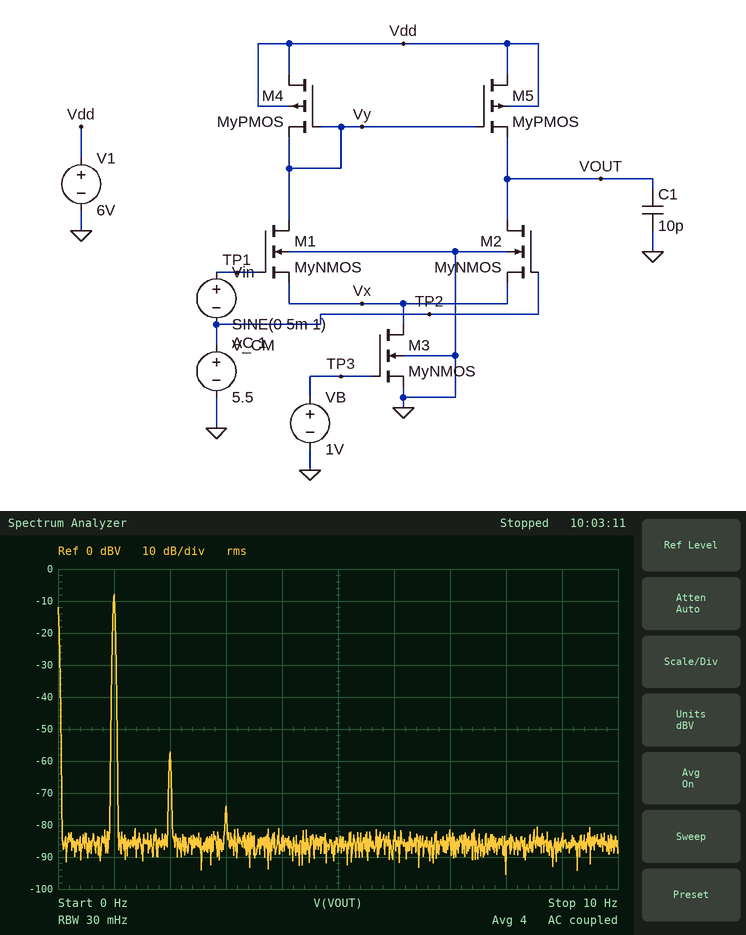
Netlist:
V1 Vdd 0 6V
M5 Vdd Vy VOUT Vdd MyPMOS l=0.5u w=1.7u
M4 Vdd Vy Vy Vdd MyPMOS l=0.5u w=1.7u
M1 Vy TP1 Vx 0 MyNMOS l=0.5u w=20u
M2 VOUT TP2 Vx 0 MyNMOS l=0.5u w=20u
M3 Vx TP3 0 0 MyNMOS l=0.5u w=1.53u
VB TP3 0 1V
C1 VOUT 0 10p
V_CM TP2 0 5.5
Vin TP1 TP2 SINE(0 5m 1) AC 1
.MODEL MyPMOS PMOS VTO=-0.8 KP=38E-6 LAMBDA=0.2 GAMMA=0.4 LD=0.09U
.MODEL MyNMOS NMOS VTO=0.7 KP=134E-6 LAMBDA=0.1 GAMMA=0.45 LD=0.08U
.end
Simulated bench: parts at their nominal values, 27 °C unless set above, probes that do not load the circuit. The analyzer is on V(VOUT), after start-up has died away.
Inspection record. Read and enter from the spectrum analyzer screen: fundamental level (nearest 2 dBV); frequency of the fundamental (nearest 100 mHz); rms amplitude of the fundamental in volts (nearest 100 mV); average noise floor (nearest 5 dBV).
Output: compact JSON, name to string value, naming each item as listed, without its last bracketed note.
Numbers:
{"fundamental level": "-8 dBV", "frequency of the fundamental": "1.0 Hz", "rms amplitude of the fundamental in volts": "400 mV", "average noise floor": "-85 dBV"}
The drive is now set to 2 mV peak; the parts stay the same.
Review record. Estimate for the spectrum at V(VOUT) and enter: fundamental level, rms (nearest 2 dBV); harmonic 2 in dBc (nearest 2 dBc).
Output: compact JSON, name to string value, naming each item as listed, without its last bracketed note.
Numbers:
{"fundamental level, rms": "-16 dBV", "harmonic 2 in dBc": "-58 dBc"}
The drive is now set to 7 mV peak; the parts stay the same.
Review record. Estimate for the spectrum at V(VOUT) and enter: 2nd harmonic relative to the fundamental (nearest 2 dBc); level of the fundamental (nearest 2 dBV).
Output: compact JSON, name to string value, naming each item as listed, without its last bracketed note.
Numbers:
{"2nd harmonic relative to the fundamental": "-28 dBc", "level of the fundamental": "-6 dBV"}
